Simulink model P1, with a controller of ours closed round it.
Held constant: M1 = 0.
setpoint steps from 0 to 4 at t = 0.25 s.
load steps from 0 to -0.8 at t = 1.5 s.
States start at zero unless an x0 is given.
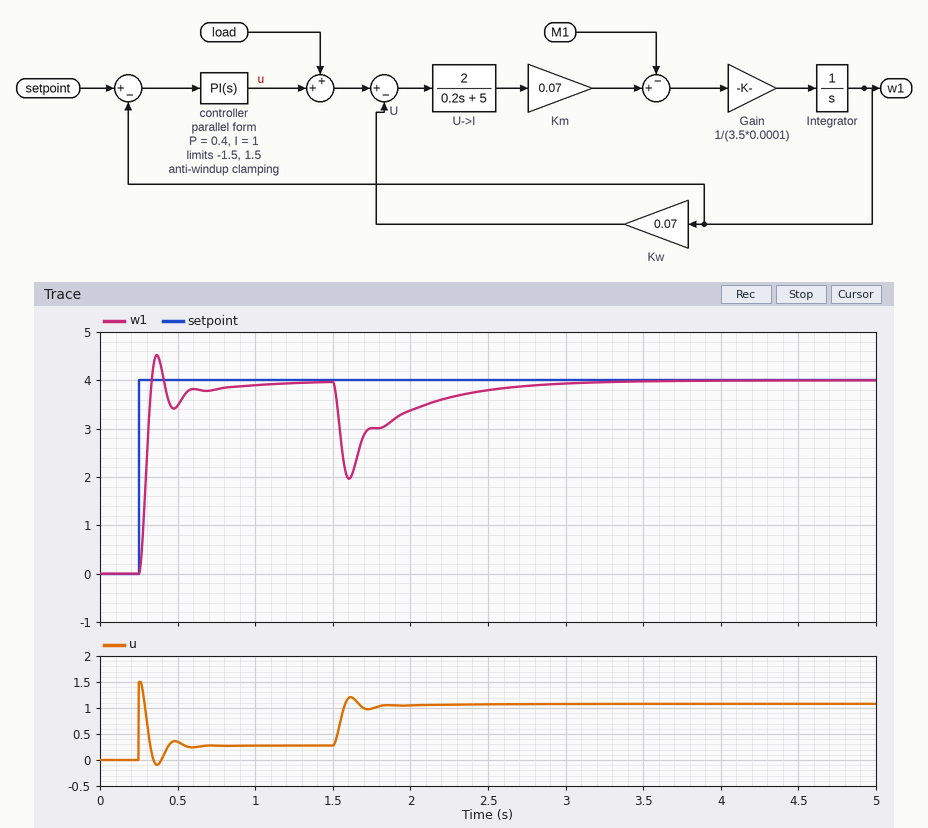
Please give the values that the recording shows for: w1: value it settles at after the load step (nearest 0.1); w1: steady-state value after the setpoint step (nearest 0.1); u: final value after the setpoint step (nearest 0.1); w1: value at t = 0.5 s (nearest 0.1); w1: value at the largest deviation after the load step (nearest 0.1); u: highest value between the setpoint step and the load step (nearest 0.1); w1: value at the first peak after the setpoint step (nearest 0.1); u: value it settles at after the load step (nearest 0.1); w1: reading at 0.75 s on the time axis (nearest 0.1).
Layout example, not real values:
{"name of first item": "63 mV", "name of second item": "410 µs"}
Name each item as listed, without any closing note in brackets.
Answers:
{"w1: value it settles at after the load step": "4.0", "w1: steady-state value after the setpoint step": "4.0", "u: final value after the setpoint step": "0.3", "w1: value at t = 0.5 s": "3.5", "w1: value at the largest deviation after the load step": "2.0", "u: highest value between the setpoint step and the load step": "1.5", "w1: value at the first peak after the setpoint step": "4.5", "u: value it settles at after the load step": "1.1", "w1: reading at 0.75 s on the time axis": "3.8"}
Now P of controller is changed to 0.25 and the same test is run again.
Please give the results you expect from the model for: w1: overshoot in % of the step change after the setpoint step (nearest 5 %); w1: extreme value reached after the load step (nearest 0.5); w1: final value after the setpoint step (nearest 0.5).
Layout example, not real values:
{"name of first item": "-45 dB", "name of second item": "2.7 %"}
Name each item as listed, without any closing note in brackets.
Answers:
{"w1: overshoot in % of the step change after the setpoint step": "10 %", "w1: extreme value reached after the load step": "1.5", "w1: final value after the setpoint step": "4.0"}
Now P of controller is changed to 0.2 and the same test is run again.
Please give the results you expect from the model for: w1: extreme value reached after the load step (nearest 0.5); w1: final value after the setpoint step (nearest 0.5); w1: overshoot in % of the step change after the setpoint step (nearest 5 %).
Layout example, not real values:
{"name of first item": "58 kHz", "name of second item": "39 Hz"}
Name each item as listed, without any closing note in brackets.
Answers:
{"w1: extreme value reached after the load step": "1.0", "w1: final value after the setpoint step": "4.0", "w1: overshoot in % of the step change after the setpoint step": "10 %"}
